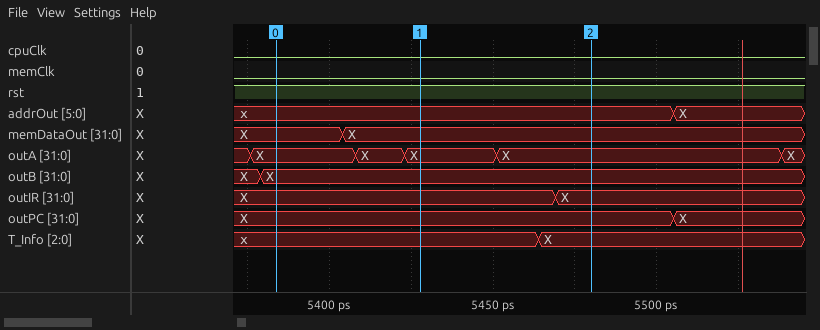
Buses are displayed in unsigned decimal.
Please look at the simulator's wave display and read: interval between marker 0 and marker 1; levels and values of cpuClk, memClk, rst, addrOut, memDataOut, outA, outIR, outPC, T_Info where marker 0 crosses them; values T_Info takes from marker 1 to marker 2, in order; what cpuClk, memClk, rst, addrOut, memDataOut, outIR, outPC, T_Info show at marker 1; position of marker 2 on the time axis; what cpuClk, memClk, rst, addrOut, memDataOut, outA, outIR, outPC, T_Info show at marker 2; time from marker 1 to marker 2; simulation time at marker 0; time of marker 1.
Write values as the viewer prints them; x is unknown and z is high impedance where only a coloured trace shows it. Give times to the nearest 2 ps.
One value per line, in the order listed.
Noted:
44 ps
cpuClk=0, memClk=0, rst=1, addrOut=x, memDataOut=X, outA=X, outIR=X, outPC=X, T_Info=x
x, X
cpuClk=0, memClk=0, rst=1, addrOut=x, memDataOut=X, outIR=X, outPC=X, T_Info=x
5480 ps
cpuClk=0, memClk=0, rst=1, addrOut=x, memDataOut=X, outA=X, outIR=X, outPC=X, T_Info=X
52 ps
5384 ps
5428 ps
